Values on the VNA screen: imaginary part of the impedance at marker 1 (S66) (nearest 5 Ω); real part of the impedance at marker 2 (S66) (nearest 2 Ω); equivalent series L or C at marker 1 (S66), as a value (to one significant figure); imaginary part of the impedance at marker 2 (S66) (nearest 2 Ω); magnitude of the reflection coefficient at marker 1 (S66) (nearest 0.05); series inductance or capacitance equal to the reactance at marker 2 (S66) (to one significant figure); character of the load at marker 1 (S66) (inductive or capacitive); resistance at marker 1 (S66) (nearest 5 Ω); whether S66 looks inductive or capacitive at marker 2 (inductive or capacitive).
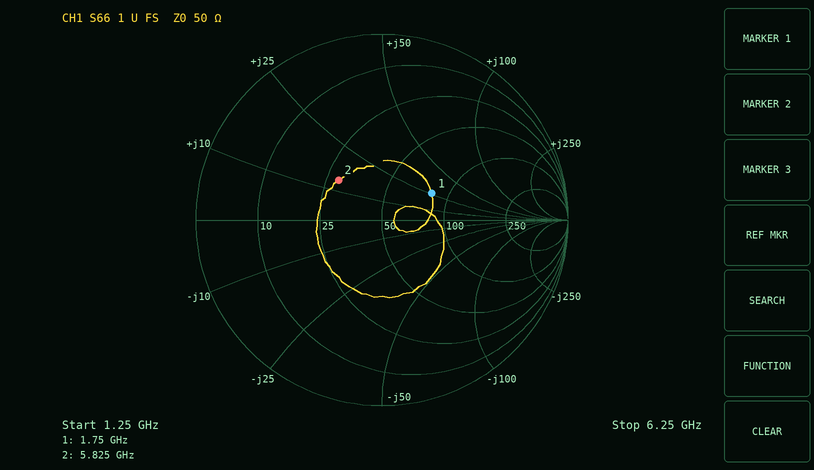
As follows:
+25 Ω
28 Ω
2 nH
+14 Ω
0.30
400 pH
inductive
80 Ω
inductive
